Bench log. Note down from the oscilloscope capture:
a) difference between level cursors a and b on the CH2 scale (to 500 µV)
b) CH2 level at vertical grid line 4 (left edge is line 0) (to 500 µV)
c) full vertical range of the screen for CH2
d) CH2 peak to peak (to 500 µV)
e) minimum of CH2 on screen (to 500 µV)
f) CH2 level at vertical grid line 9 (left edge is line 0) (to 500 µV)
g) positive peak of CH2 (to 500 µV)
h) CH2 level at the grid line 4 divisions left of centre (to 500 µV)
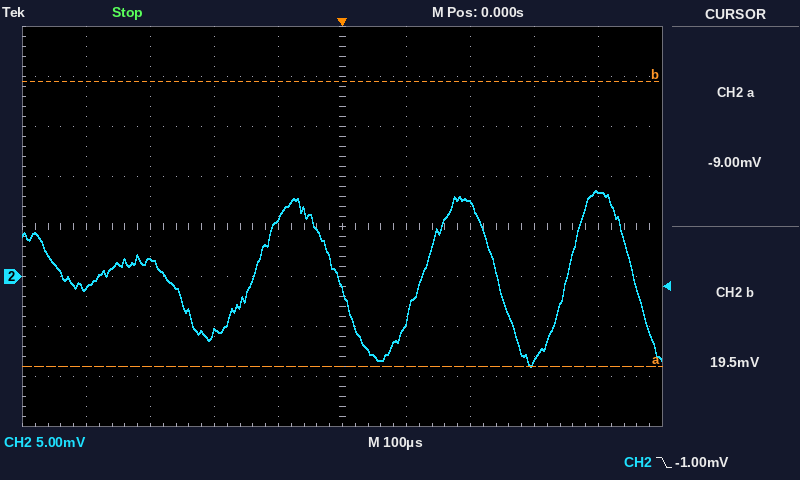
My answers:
28.5 mV
6.0 mV
40 mV
17.5 mV
-9.0 mV
8.5 mV
8.5 mV
-1.0 mV
